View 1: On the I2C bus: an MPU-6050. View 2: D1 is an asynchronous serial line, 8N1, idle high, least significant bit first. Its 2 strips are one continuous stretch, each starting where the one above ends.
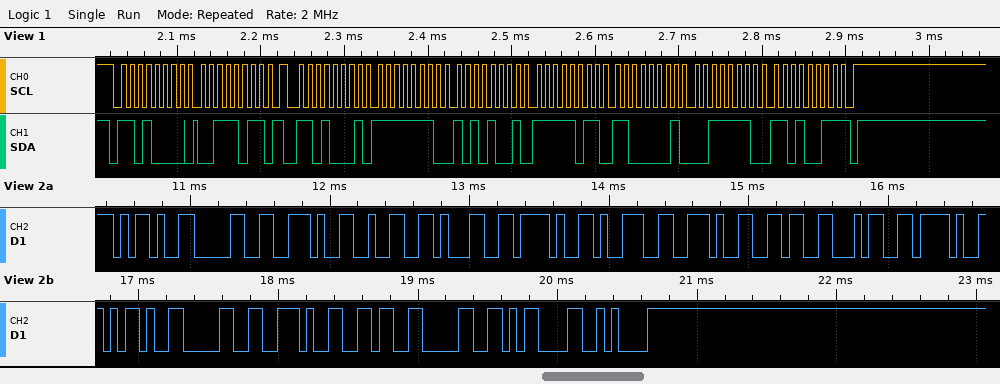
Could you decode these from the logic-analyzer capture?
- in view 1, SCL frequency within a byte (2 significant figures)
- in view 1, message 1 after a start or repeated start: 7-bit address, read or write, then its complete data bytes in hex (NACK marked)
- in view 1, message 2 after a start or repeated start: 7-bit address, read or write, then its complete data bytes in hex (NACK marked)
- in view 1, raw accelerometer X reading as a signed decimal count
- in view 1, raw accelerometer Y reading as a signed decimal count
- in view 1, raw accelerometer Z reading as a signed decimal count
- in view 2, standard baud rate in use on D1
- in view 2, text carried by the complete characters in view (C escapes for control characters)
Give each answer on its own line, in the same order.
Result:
100 kHz
0x68 write: 3B
0x68 read: FE A9 FB C1 3E D3 NACK
-343
-1087
16083
19200 baud
"-0.21/9.64/-0.60\r\n"
